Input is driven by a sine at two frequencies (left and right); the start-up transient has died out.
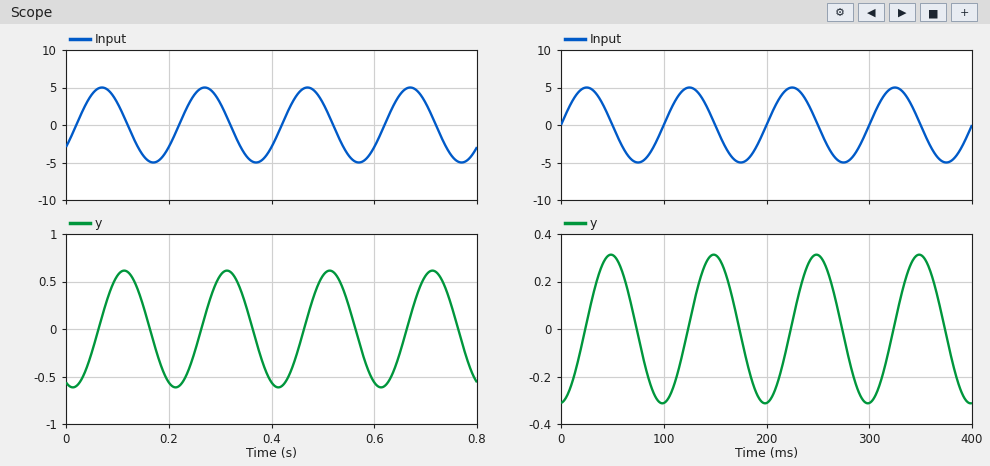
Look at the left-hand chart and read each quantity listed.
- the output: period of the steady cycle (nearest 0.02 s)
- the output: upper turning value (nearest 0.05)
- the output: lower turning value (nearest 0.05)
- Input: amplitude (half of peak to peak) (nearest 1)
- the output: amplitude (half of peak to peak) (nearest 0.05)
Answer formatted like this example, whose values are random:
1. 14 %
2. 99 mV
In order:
1. 0.20 s
2. 0.60
3. -0.60
4. 5
5. 0.60
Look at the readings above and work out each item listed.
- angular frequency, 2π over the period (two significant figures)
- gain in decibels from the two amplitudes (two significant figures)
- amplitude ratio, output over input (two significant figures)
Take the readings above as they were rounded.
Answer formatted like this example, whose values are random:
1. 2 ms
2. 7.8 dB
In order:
1. 31 rad/s
2. -18 dB
3. 0.12
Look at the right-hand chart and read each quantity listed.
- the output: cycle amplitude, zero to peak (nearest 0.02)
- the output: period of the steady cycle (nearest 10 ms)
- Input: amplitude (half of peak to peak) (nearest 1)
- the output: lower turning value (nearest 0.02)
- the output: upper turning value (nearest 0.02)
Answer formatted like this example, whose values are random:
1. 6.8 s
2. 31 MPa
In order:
1. 0.32
2. 100 ms
3. 5
4. -0.32
5. 0.32
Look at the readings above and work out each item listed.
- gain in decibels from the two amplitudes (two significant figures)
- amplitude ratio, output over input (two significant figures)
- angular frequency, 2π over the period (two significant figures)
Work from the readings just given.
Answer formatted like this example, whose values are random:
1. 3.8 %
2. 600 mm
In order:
1. -24 dB
2. 0.064
3. 0.063 rad/ms
